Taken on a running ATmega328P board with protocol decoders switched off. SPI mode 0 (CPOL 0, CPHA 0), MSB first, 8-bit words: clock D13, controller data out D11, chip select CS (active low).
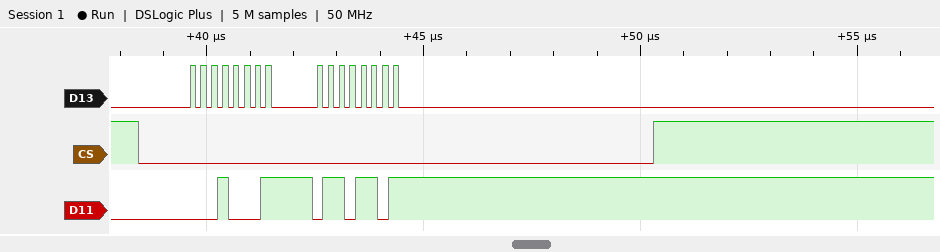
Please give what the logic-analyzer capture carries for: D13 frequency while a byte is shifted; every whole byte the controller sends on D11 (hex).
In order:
4 MHz
11 6D
